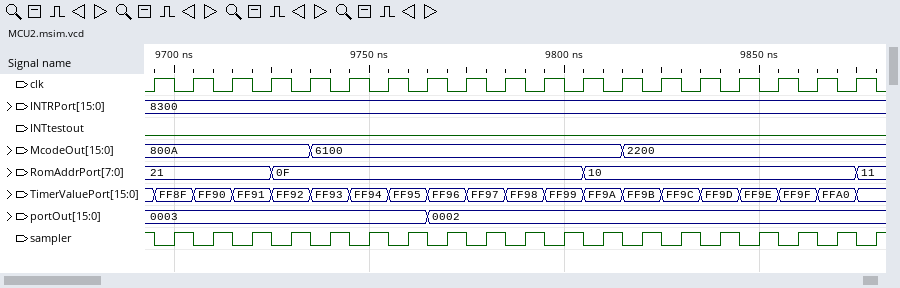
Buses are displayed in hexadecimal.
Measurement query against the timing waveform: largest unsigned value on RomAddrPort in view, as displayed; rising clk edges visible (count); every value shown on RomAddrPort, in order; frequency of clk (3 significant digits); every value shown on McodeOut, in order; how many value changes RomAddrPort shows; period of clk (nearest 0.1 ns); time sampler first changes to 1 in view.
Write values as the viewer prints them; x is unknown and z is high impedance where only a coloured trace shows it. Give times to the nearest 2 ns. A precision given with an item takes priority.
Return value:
21
19
21, 0F, 10, 11
100 MHz
800A, 6100, 2200
3
10 ns
9700 ns
